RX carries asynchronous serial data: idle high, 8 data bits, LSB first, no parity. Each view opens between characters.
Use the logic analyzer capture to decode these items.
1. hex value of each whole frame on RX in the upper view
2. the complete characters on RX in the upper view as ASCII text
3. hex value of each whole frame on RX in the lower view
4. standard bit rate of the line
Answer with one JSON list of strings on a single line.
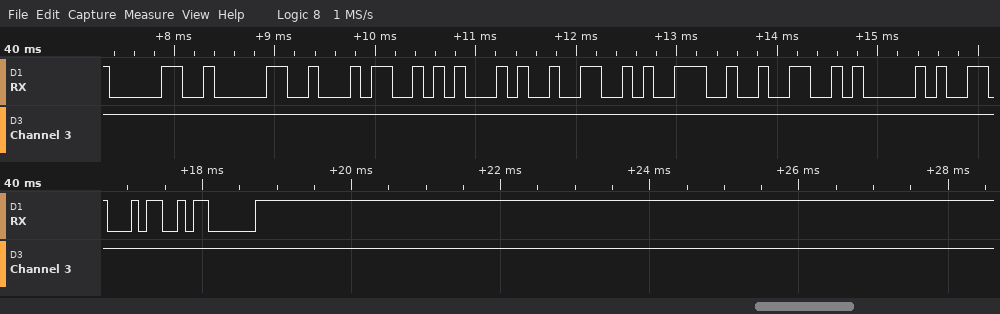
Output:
["30, 30, 34, 45, 32, 39, 32, 41", "\"004E292A\"", "34, 03", "9600 baud"]
